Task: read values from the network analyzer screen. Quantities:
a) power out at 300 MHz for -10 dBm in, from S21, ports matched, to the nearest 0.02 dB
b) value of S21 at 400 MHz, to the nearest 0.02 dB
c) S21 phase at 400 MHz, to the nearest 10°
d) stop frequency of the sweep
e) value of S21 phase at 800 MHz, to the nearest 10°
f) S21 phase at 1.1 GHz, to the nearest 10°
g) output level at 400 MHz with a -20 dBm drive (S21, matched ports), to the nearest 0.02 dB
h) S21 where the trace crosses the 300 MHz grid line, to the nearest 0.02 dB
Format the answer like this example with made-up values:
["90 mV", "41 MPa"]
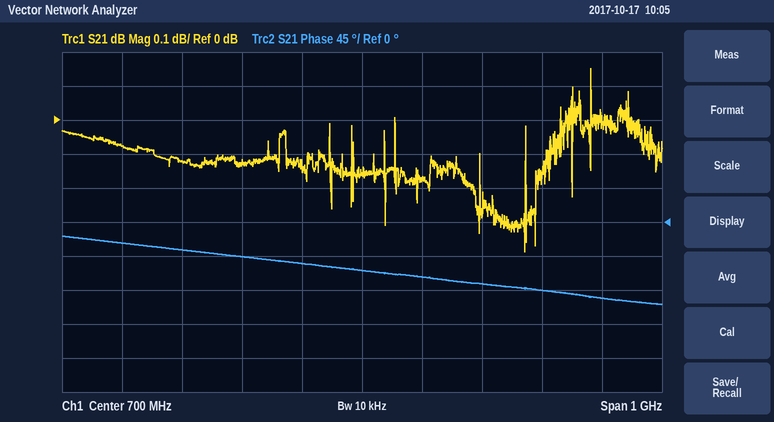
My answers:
["-10.08 dBm", "-0.12 dB", "-40°", "1.2 GHz", "-70°", "-100°", "-20.12 dBm", "-0.08 dB"]
